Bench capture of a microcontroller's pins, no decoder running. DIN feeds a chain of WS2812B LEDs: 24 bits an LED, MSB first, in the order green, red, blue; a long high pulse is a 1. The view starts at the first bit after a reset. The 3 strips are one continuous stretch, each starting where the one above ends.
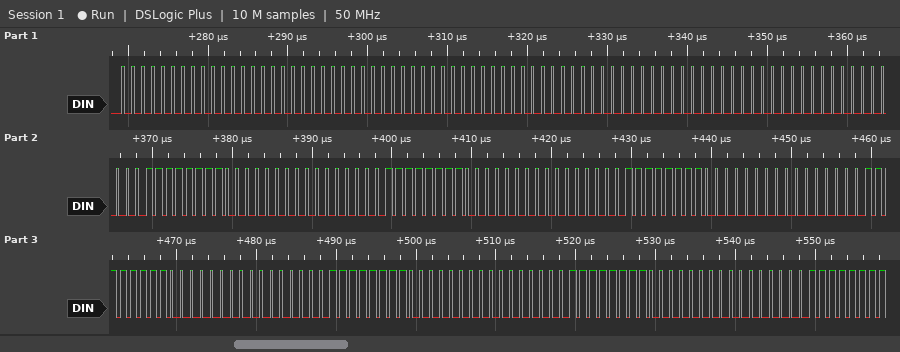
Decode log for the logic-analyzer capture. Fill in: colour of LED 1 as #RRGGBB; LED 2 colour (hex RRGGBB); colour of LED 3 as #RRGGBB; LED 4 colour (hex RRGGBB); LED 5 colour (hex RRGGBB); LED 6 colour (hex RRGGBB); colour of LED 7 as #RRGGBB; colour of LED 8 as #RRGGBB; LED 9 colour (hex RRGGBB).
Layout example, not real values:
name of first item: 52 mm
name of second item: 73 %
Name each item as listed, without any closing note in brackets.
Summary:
colour of LED 1 as #RRGGBB: #000000
LED 2 colour: #000000
colour of LED 3 as #RRGGBB: #000000
LED 4 colour: #FF0000
LED 5 colour: #FF0000
LED 6 colour: #FF0000
colour of LED 7 as #RRGGBB: #FF0000
colour of LED 8 as #RRGGBB: #FF0000
LED 9 colour: #FF0000
